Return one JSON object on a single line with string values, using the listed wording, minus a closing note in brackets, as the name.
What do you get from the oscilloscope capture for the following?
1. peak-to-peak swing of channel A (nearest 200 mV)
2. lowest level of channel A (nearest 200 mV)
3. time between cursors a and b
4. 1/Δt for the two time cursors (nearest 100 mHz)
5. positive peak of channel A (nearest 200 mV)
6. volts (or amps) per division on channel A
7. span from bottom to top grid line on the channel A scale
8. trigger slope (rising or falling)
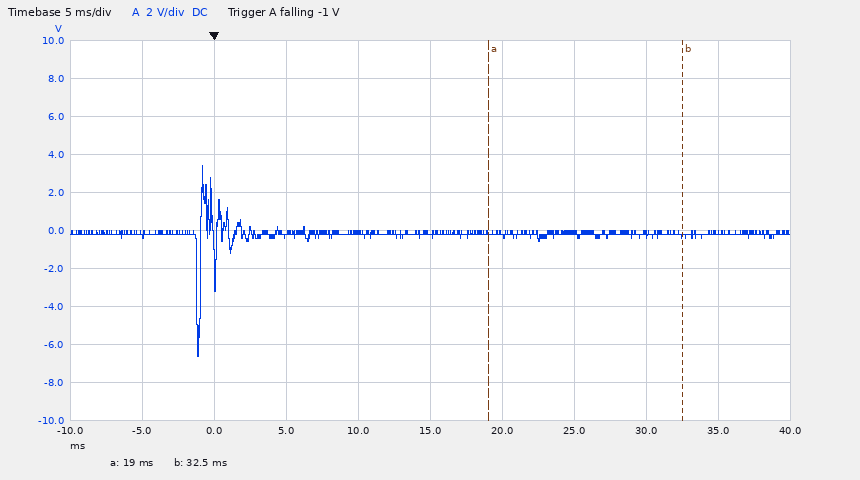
{"peak-to-peak swing of channel A": "10.0 V", "lowest level of channel A": "-6.6 V", "time between cursors a and b": "13.5 ms", "1/Δt for the two time cursors": "74.1 Hz", "positive peak of channel A": "3.4 V", "volts (or amps) per division on channel A": "2 V", "span from bottom to top grid line on the channel A scale": "20 V", "trigger slope": "falling"}
